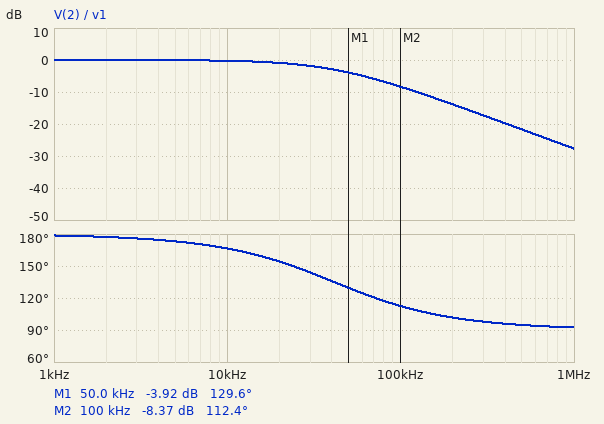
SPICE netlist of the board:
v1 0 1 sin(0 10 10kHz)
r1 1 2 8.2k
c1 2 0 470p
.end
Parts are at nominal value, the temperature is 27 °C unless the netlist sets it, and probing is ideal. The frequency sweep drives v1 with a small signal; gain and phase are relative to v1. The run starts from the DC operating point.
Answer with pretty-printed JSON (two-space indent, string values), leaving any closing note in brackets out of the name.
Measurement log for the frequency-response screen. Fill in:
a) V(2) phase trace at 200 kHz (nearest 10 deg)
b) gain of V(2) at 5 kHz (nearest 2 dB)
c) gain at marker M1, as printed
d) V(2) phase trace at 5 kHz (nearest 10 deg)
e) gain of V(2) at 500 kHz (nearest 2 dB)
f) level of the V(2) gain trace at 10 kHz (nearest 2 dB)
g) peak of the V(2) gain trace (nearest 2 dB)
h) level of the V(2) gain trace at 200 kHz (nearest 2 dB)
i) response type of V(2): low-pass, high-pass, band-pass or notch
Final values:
{
  "V(2) phase trace at 200 kHz": "100 deg",
  "gain of V(2) at 5 kHz": "0 dB",
  "gain at marker M1, as printed": "-3.92 dB",
  "V(2) phase trace at 5 kHz": "170 deg",
  "gain of V(2) at 500 kHz": "-22 dB",
  "level of the V(2) gain trace at 10 kHz": "0 dB",
  "peak of the V(2) gain trace": "0 dB",
  "level of the V(2) gain trace at 200 kHz": "-14 dB",
  "response type of V(2): low-pass, high-pass, band-pass or notch": "low-pass"
}
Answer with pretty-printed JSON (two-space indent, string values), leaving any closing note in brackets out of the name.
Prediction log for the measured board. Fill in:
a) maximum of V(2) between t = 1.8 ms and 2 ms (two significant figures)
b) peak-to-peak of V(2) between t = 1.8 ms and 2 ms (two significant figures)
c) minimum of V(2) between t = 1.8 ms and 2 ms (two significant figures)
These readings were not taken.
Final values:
{
  "maximum of V(2) between t = 1.8 ms and 2 ms": "9.7 V",
  "peak-to-peak of V(2) between t = 1.8 ms and 2 ms": "19 V",
  "minimum of V(2) between t = 1.8 ms and 2 ms": "-9.7 V"
}
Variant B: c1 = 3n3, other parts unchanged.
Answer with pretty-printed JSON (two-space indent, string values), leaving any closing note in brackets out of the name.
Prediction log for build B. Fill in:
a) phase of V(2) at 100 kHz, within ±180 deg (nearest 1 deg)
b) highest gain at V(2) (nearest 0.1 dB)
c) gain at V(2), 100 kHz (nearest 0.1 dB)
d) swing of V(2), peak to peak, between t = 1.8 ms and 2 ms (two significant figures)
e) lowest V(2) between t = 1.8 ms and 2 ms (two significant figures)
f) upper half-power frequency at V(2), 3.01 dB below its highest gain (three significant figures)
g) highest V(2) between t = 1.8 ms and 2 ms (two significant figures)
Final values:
{
  "phase of V(2) at 100 kHz, within ±180 deg": "93 deg",
  "highest gain at V(2)": "0 dB",
  "gain at V(2), 100 kHz": "-24.6 dB",
  "swing of V(2), peak to peak, between t = 1.8 ms and 2 ms": "10 V",
  "lowest V(2) between t = 1.8 ms and 2 ms": "-5.1 V",
  "upper half-power frequency at V(2), 3.01 dB below its highest gain": "5.88 kHz",
  "highest V(2) between t = 1.8 ms and 2 ms": "5.1 V"
}
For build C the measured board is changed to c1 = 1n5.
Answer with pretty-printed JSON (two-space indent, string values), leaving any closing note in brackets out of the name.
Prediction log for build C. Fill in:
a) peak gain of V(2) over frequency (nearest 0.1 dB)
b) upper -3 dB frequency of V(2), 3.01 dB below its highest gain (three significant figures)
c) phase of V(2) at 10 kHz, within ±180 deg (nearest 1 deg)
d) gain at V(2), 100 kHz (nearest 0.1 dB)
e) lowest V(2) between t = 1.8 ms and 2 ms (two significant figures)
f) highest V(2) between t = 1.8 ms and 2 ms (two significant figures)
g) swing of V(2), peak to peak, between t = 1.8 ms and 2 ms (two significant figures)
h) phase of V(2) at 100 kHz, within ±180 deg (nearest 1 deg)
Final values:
{
  "peak gain of V(2) over frequency": "0 dB",
  "upper -3 dB frequency of V(2), 3.01 dB below its highest gain": "12.9 kHz",
  "phase of V(2) at 10 kHz, within ±180 deg": "142 deg",
  "gain at V(2), 100 kHz": "-17.8 dB",
  "lowest V(2) between t = 1.8 ms and 2 ms": "-7.9 V",
  "highest V(2) between t = 1.8 ms and 2 ms": "7.9 V",
  "swing of V(2), peak to peak, between t = 1.8 ms and 2 ms": "16 V",
  "phase of V(2) at 100 kHz, within ±180 deg": "97 deg"
}
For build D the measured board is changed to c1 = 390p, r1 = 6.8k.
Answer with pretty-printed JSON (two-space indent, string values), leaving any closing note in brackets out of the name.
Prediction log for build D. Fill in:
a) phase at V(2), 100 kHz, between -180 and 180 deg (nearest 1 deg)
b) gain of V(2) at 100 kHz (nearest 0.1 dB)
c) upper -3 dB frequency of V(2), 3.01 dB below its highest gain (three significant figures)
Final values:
{
  "phase at V(2), 100 kHz, between -180 and 180 deg": "121 deg",
  "gain of V(2) at 100 kHz": "-5.8 dB",
  "upper -3 dB frequency of V(2), 3.01 dB below its highest gain": "60.0 kHz"
}
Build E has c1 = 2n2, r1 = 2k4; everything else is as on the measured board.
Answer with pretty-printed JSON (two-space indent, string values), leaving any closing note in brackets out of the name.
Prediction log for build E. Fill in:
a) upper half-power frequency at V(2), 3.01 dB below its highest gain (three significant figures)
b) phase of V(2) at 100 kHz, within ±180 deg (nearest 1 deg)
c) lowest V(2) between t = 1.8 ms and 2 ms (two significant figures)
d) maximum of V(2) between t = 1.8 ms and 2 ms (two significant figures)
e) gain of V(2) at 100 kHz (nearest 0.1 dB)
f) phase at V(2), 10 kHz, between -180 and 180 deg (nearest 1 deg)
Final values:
{
  "upper half-power frequency at V(2), 3.01 dB below its highest gain": "30.1 kHz",
  "phase of V(2) at 100 kHz, within ±180 deg": "107 deg",
  "lowest V(2) between t = 1.8 ms and 2 ms": "-9.5 V",
  "maximum of V(2) between t = 1.8 ms and 2 ms": "9.5 V",
  "gain of V(2) at 100 kHz": "-10.8 dB",
  "phase at V(2), 10 kHz, between -180 and 180 deg": "162 deg"
}
